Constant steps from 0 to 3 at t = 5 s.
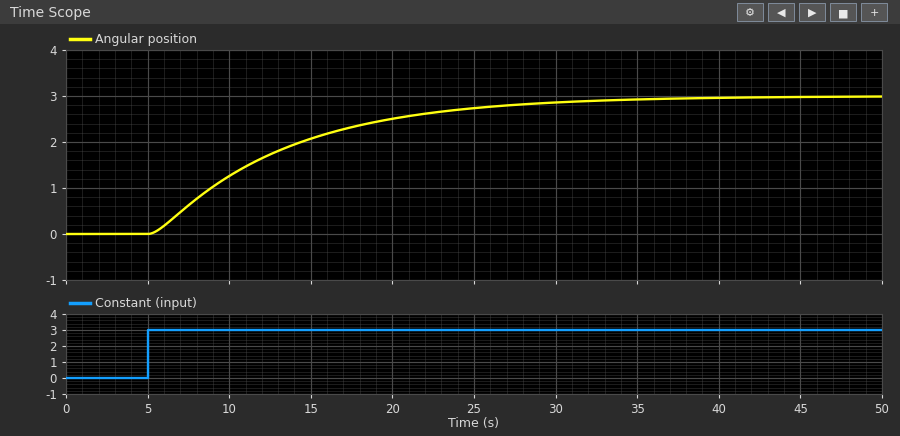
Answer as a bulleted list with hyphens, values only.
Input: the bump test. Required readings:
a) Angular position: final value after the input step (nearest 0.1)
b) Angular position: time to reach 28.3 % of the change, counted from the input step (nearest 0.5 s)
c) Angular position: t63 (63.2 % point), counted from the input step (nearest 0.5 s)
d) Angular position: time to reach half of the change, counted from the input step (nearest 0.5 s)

- 3.0
- 3.5 s
- 8.5 s
- 6.0 s
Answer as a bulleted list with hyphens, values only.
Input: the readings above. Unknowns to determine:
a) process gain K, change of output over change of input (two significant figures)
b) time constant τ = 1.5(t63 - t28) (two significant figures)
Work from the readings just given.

- 1.0
- 7.5 s
